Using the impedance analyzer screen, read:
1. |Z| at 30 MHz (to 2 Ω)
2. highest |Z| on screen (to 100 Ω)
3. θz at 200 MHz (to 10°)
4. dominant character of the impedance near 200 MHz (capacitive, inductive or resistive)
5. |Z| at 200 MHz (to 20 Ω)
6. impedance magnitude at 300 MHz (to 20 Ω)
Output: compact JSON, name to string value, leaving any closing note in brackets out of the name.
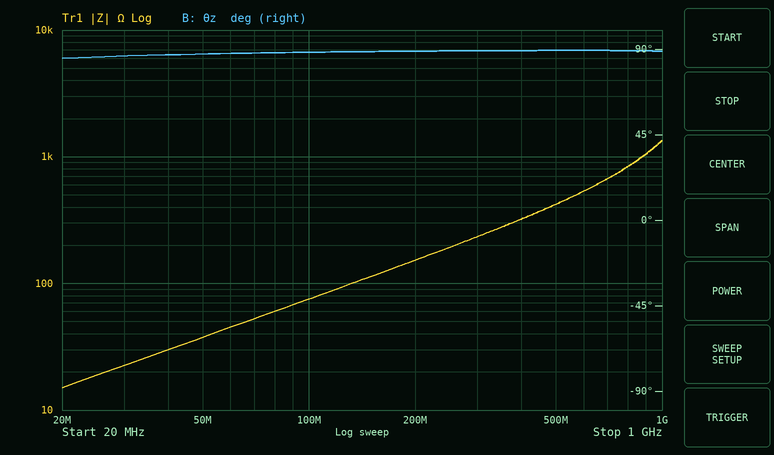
{"|Z| at 30 MHz": "22 Ω", "highest |Z| on screen": "1.3 kΩ", "θz at 200 MHz": "90°", "dominant character of the impedance near 200 MHz": "inductive", "|Z| at 200 MHz": "160 Ω", "impedance magnitude at 300 MHz": "240 Ω"}
